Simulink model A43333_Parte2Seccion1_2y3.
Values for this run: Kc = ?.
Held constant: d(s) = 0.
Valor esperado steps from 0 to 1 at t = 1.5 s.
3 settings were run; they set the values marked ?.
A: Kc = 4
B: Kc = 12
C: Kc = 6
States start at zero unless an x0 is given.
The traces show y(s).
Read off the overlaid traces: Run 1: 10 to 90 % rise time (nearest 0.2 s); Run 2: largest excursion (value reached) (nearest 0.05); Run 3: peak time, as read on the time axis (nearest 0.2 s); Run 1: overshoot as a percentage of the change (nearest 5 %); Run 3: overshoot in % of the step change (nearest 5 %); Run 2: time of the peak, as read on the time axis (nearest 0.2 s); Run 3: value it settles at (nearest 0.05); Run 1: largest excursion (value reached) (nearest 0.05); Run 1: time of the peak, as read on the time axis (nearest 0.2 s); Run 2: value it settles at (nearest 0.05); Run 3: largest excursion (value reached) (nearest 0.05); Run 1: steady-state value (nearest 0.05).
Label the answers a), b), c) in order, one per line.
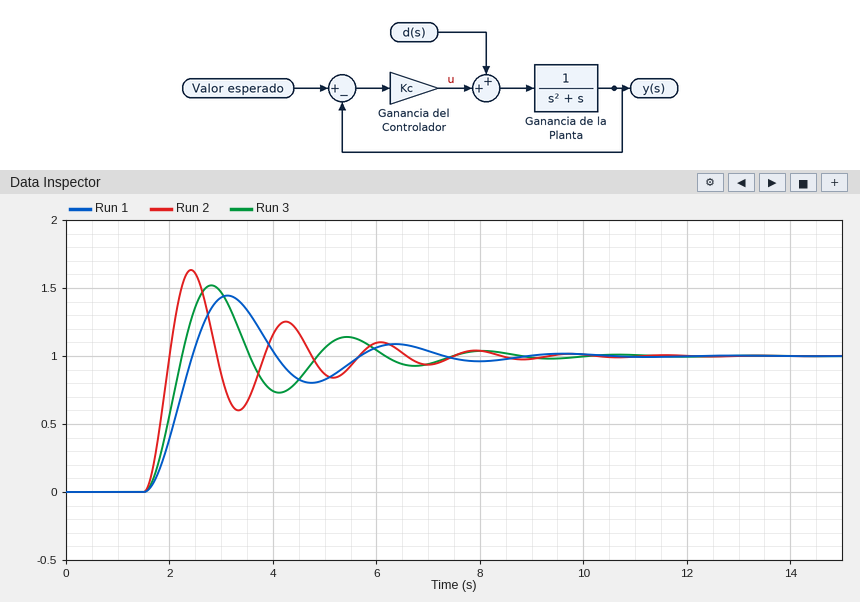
a) 0.6 s
b) 1.65
c) 2.8 s
d) 45 %
e) 50 %
f) 2.4 s
g) 1.00
h) 1.45
i) 3.2 s
j) 1.00
k) 1.50
l) 1.00
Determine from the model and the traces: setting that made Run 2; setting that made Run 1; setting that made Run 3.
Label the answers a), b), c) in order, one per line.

a) B
b) A
c) C
